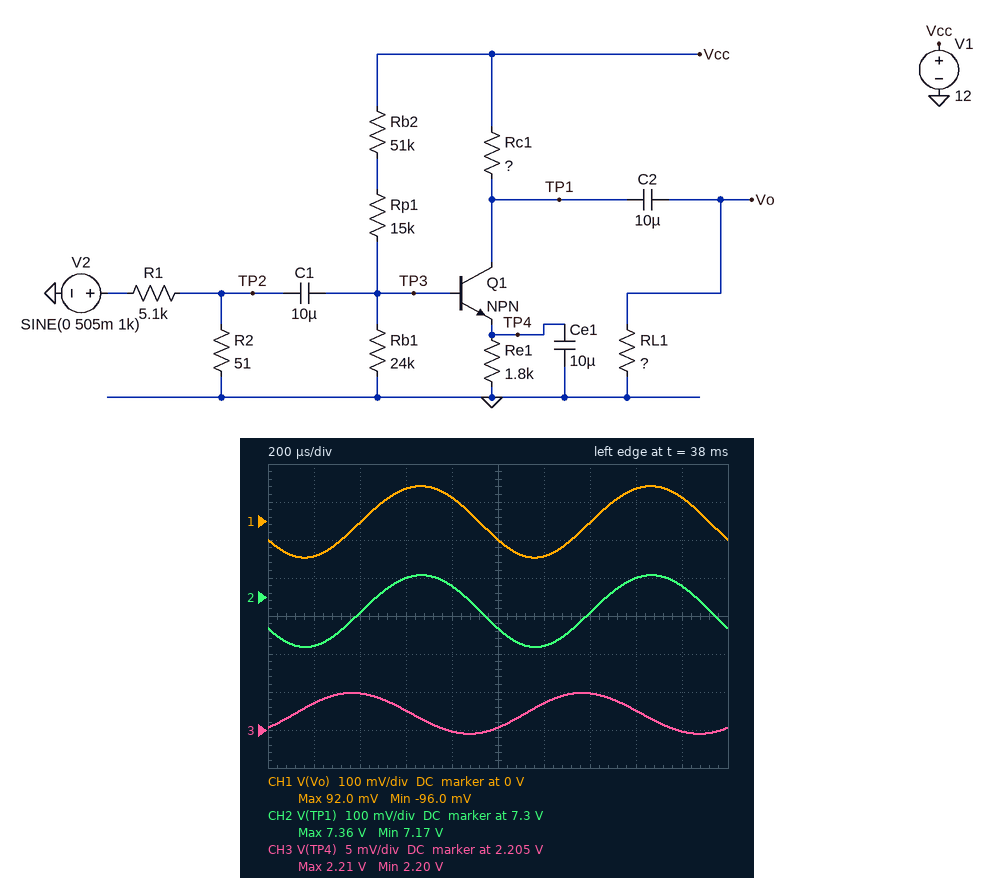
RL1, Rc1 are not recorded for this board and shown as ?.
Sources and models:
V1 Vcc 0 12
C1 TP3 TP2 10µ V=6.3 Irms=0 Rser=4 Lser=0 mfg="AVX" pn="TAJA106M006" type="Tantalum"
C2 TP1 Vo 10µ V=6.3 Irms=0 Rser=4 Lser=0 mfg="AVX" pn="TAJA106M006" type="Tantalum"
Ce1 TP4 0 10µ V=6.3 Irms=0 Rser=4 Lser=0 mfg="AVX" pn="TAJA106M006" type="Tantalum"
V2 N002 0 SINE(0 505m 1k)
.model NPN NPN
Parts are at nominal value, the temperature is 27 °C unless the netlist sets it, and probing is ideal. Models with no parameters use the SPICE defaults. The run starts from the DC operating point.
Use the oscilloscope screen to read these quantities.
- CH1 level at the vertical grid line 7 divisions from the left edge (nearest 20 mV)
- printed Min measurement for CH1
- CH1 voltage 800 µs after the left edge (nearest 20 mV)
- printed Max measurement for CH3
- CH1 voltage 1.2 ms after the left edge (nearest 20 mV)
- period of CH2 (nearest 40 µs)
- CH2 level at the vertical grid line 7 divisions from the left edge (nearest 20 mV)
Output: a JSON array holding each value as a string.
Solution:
["0 V", "-96.0 mV", "60 mV", "2.21 V", "-100 mV", "1.00 ms", "7.26 V"]
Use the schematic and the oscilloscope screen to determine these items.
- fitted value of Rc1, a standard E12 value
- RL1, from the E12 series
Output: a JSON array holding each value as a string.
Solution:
["3.9 kΩ", "680 Ω"]
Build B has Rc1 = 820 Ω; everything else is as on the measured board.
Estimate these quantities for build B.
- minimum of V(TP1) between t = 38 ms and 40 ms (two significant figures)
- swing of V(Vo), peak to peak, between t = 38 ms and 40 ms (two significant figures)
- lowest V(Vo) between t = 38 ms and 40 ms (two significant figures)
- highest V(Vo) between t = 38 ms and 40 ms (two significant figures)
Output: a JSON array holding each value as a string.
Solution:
["11 V", "120 mV", "-62 mV", "59 mV"]
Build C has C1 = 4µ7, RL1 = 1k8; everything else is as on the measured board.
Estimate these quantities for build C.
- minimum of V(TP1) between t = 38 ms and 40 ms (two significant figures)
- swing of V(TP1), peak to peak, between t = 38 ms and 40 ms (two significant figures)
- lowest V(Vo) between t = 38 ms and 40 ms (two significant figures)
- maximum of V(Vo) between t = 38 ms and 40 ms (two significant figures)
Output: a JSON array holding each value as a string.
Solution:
["7.1 V", "400 mV", "-200 mV", "190 mV"]
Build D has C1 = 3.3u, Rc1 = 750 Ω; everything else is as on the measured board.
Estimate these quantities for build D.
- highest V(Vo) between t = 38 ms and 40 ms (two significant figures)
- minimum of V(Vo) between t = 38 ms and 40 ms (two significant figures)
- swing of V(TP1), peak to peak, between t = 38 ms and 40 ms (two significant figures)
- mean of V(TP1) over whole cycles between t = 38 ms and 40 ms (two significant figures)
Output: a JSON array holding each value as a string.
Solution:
["56 mV", "-59 mV", "120 mV", "11 V"]
